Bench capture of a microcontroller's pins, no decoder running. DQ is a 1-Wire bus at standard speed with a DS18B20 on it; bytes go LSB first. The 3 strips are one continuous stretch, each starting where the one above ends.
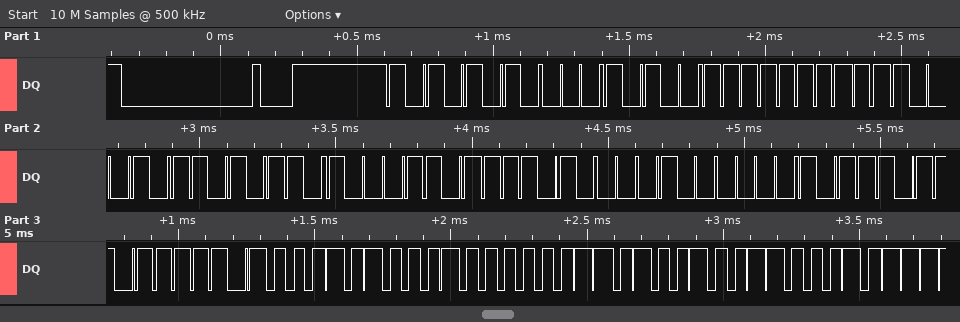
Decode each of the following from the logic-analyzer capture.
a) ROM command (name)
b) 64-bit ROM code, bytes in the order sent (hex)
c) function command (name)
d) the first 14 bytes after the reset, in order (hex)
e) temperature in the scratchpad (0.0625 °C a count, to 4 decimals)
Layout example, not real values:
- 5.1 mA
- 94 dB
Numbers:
- Match ROM
- 28 FF 47 6B B1 17 02 DD
- Read Scratchpad
- 55 28 FF 47 6B B1 17 02 DD BE 28 02 4B 46
- 34.5000 °C
